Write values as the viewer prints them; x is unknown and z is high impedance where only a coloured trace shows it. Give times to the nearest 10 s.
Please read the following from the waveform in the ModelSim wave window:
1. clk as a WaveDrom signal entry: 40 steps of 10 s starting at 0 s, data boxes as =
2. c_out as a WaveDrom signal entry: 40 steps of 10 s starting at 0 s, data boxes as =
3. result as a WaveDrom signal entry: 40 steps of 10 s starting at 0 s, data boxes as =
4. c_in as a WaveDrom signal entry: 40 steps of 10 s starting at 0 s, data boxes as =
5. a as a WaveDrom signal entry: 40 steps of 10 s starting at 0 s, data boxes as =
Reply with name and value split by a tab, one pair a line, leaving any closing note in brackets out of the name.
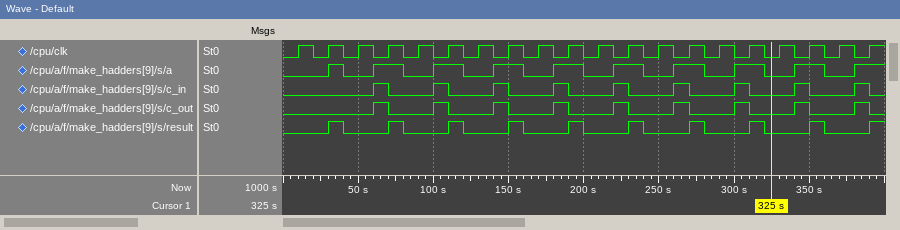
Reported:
clk as a WaveDrom signal entry: 40 steps of 10 s starting at 0 s, data boxes as =	{name: 'clk', wave: '0101010101010101010101010101010101010101'}
c_out as a WaveDrom signal entry: 40 steps of 10 s starting at 0 s, data boxes as =	{name: 'c_out', wave: '0.....10..10..10..10..10..10..10..10..10'}
result as a WaveDrom signal entry: 40 steps of 10 s starting at 0 s, data boxes as =	{name: 'result', wave: '0..10..10..10..10..10..10..10..10..10..1'}
c_in as a WaveDrom signal entry: 40 steps of 10 s starting at 0 s, data boxes as =	{name: 'c_in', wave: '0.....10..10..10..10..10..10..10..10..10'}
a as a WaveDrom signal entry: 40 steps of 10 s starting at 0 s, data boxes as =	{name: 'a', wave: '0..10.1.0.1.0.1.0.1.0.1.0.1.0.1.0.1.0.1.'}
